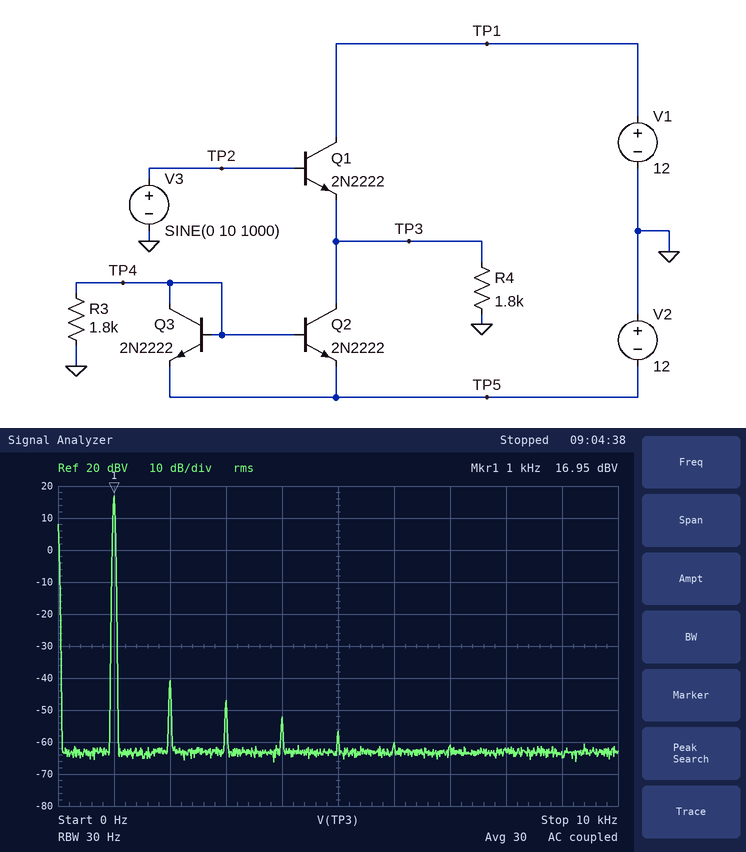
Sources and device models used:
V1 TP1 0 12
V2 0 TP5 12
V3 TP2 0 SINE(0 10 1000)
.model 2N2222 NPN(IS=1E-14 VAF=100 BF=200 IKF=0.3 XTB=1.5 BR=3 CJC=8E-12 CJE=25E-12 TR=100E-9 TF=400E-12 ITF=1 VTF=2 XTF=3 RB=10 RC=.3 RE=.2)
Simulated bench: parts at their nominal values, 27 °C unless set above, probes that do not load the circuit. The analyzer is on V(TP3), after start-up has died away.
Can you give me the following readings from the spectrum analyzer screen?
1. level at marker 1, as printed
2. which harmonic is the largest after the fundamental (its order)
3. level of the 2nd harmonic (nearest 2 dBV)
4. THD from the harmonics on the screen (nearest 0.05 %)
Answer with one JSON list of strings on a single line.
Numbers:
["16.95 dBV", "2", "-40 dBV", "0.15 %"]
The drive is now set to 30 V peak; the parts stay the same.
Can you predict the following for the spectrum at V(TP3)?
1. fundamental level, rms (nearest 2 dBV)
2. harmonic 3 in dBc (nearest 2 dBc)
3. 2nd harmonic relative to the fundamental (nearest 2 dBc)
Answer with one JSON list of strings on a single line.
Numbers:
["20 dBV", "-12 dBc", "-28 dBc"]
